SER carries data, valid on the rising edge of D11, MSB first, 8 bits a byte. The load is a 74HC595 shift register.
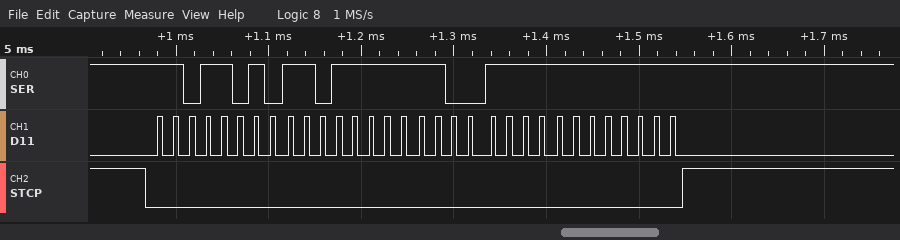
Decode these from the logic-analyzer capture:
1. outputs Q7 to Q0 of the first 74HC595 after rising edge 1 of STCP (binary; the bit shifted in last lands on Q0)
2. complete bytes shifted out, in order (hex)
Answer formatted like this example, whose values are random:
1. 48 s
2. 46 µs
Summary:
1. 11111111
2. DA DF CF FF
